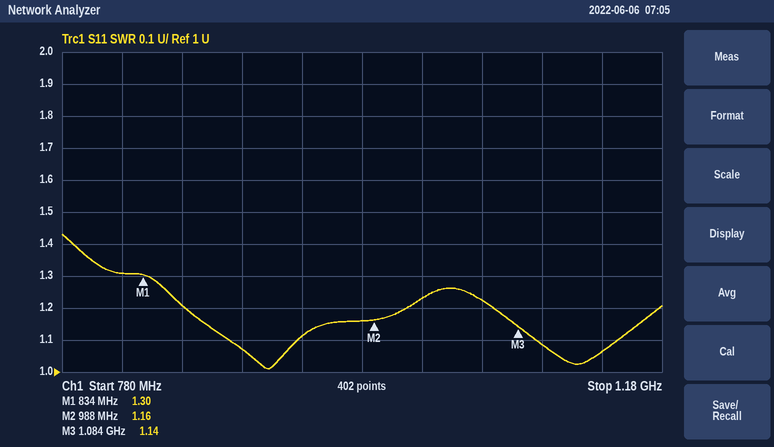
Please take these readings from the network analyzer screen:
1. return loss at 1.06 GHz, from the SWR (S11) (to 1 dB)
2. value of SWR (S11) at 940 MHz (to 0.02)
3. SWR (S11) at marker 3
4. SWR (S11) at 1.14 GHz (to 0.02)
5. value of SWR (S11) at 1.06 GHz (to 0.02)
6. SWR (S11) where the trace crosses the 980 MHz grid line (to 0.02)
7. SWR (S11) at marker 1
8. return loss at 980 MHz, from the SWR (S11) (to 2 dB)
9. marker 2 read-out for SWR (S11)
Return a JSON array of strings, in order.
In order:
["20 dB", "1.12", "1.14", "1.06", "1.22", "1.16", "1.30", "22 dB", "1.16"]
